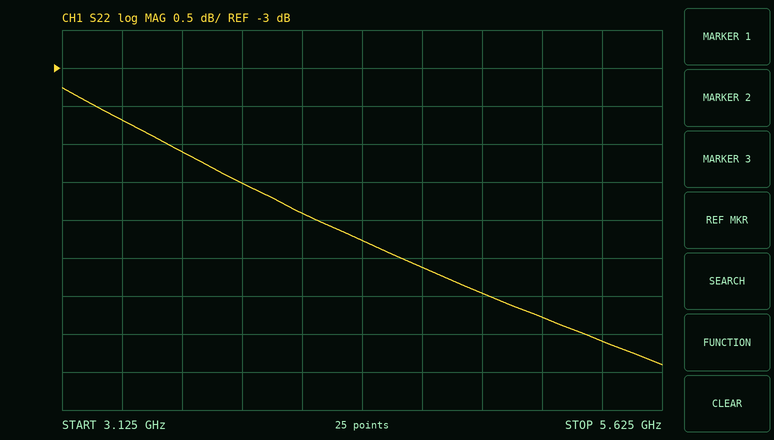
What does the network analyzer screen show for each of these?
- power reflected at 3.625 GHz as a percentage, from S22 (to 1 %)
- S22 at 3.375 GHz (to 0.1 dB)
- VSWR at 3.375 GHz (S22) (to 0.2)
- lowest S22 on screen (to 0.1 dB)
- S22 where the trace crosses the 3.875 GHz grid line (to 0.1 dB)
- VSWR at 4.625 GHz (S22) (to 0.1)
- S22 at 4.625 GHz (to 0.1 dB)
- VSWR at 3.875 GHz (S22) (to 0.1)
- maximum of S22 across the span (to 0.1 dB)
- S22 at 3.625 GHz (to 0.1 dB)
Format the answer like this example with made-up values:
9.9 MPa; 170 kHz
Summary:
39 %; -3.7 dB; 4.8; -6.9 dB; -4.5 dB; 3.2; -5.6 dB; 3.9; -3.3 dB; -4.1 dB
